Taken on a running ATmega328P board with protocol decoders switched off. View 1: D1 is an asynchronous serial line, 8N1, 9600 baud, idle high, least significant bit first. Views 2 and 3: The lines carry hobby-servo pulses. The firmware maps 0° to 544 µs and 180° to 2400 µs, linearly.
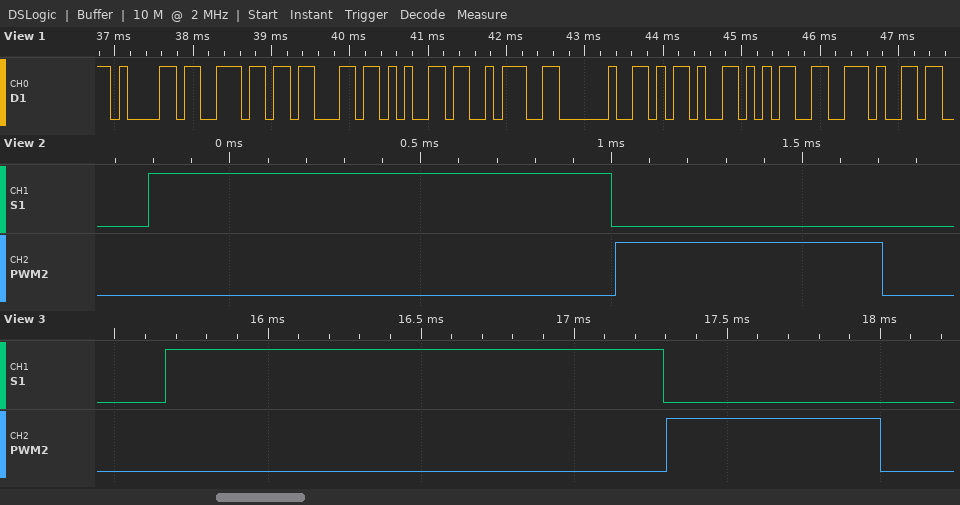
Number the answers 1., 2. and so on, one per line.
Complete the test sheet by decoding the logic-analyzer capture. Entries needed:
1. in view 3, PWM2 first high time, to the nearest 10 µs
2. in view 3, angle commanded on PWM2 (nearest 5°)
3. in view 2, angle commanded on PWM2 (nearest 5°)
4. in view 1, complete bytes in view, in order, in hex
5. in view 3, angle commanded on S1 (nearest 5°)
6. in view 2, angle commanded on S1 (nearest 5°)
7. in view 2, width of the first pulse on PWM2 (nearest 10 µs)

1. 700 µs
2. 15°
3. 15°
4. 0x61 0x6E 0x63 0x65 0x3A 0x20 0x2D 0x35 0x2E
5. 105°
6. 65°
7. 700 µs
